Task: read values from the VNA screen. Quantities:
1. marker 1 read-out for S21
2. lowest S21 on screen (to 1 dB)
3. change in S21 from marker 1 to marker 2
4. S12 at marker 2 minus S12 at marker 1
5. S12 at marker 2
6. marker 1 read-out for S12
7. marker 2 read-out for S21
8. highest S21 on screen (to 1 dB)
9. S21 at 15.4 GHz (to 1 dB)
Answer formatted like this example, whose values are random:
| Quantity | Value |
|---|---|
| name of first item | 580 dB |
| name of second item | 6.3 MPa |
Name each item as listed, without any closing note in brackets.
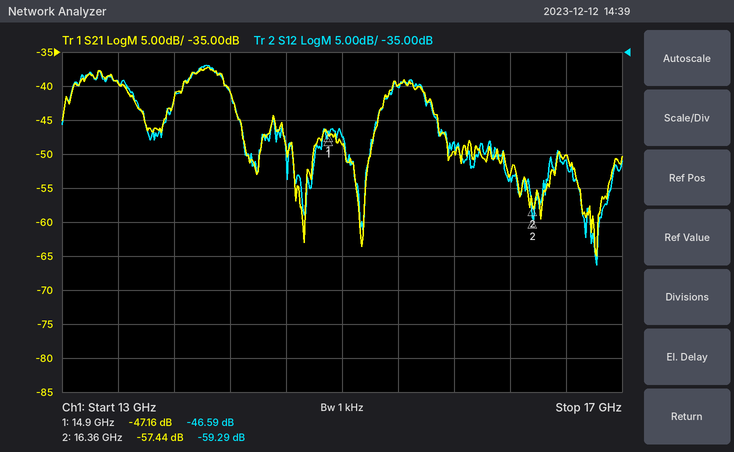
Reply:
| Quantity | Value |
|---|---|
| marker 1 read-out for S21 | -47.16 dB |
| lowest S21 on screen | -65 dB |
| change in S21 from marker 1 to marker 2 | -10.28 dB |
| S12 at marker 2 minus S12 at marker 1 | -12.70 dB |
| S12 at marker 2 | -59.29 dB |
| marker 1 read-out for S12 | -46.59 dB |
| marker 2 read-out for S21 | -57.44 dB |
| highest S21 on screen | -37 dB |
| S21 at 15.4 GHz | -40 dB |
